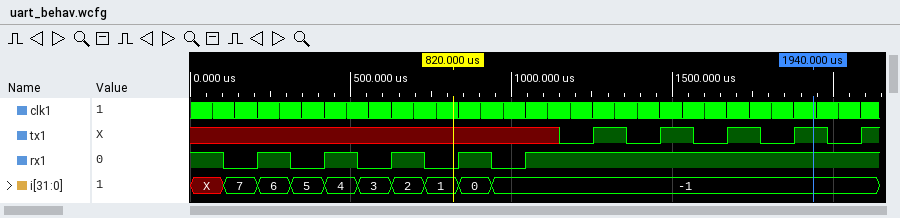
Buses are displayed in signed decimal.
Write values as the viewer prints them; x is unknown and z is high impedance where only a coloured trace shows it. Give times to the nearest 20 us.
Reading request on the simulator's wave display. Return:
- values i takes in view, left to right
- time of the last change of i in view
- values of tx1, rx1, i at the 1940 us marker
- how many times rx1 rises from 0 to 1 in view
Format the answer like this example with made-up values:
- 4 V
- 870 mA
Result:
- X, 7, 6, 5, 4, 3, 2, 1, 0, -1
- 940 us
- tx1=1, rx1=1, i=-1
- 5
